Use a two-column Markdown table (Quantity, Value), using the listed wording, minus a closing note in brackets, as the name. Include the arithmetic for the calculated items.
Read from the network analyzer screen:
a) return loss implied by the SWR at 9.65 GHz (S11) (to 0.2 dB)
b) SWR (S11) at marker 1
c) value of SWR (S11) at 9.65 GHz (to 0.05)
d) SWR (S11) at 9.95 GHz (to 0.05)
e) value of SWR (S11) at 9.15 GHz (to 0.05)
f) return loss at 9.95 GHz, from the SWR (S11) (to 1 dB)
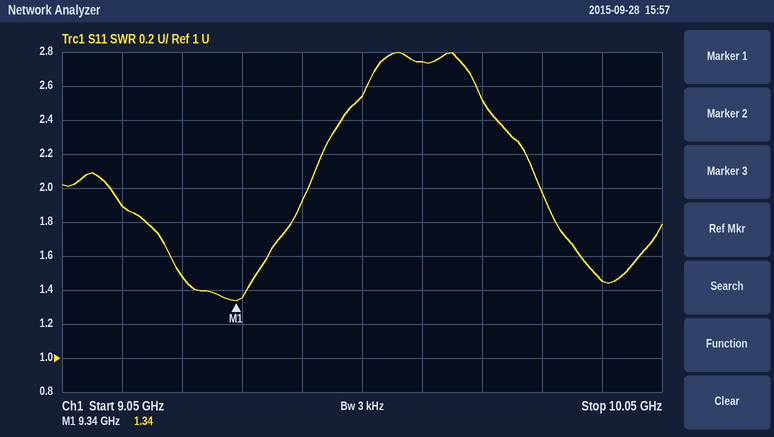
| Quantity | Value |
|---|---|
| return loss implied by the SWR at 9.65 GHz (S11) | −20 log10((2.75 − 1)/(2.75 + 1)) ≈ 6.6 dB |
| SWR (S11) at marker 1 | 1.34 |
| value of SWR (S11) at 9.65 GHz | 2.75 |
| SWR (S11) at 9.95 GHz | 1.45 |
| value of SWR (S11) at 9.15 GHz | 1.90 |
| return loss at 9.95 GHz, from the SWR (S11) | −20 log10((1.45 − 1)/(1.45 + 1)) ≈ 15 dB |
